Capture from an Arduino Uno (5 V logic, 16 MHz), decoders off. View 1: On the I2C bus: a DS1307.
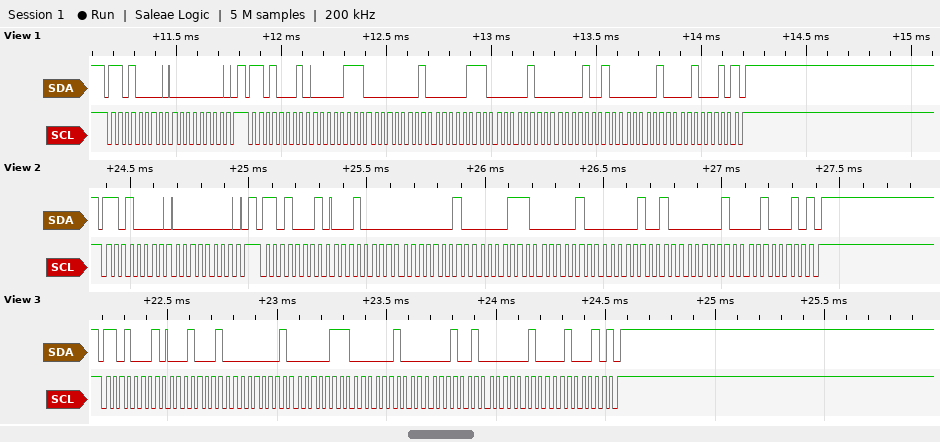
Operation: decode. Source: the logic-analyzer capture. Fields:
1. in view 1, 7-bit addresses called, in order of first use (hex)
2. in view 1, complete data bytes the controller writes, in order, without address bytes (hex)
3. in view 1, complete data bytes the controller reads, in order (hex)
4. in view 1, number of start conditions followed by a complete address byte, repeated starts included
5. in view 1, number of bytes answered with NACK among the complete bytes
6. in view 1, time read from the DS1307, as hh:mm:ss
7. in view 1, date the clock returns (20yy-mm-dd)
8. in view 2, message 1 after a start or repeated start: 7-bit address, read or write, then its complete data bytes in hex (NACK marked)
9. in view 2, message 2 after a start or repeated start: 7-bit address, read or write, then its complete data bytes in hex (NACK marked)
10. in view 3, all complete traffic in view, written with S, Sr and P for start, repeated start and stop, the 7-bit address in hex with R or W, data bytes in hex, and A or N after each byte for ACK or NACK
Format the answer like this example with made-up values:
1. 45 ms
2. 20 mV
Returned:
1. 0x68
2. 00
3. 07 01 07 04 09 02 22
4. 2
5. 1
6. 07:01:07
7. 2022-02-09
8. 0x68 write: 00
9. 0x68 read: 10 01 07 04 09 02 22 NACK
10. S 68R A 11 A 01 A 07 A 04 A 09 A 02 A 22 N P
